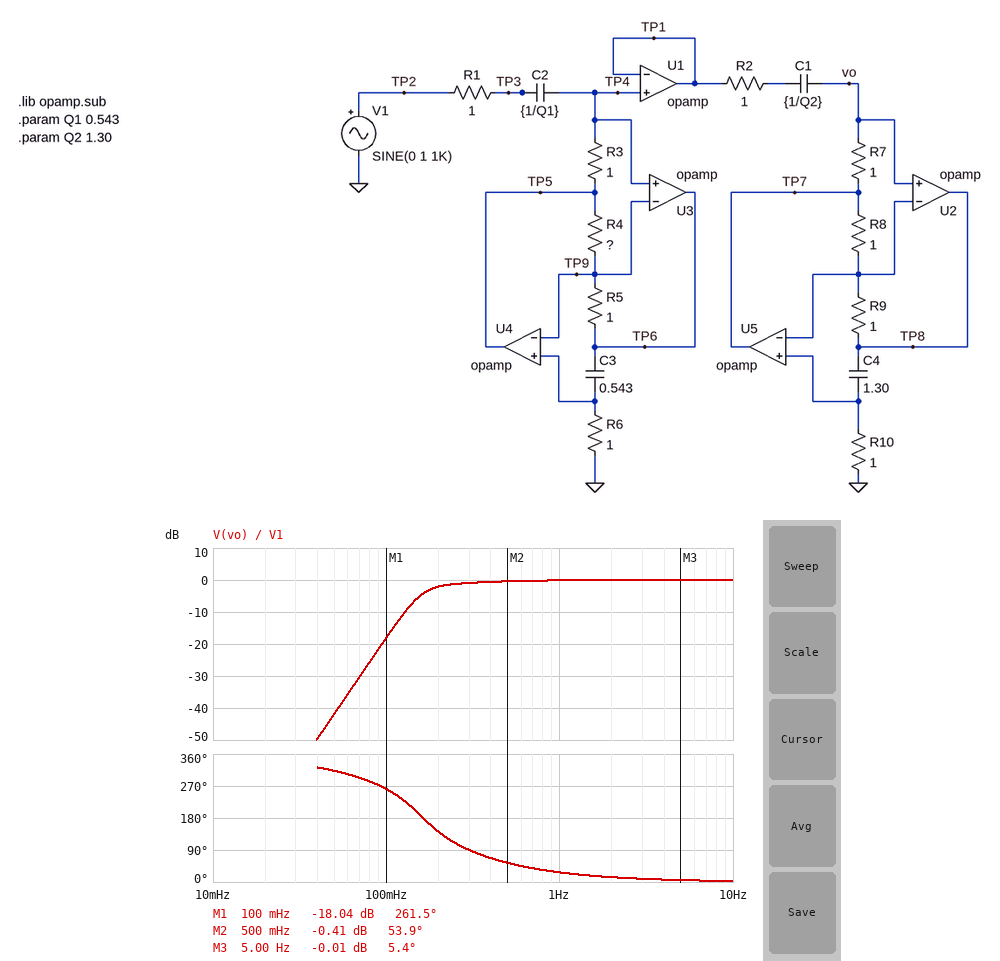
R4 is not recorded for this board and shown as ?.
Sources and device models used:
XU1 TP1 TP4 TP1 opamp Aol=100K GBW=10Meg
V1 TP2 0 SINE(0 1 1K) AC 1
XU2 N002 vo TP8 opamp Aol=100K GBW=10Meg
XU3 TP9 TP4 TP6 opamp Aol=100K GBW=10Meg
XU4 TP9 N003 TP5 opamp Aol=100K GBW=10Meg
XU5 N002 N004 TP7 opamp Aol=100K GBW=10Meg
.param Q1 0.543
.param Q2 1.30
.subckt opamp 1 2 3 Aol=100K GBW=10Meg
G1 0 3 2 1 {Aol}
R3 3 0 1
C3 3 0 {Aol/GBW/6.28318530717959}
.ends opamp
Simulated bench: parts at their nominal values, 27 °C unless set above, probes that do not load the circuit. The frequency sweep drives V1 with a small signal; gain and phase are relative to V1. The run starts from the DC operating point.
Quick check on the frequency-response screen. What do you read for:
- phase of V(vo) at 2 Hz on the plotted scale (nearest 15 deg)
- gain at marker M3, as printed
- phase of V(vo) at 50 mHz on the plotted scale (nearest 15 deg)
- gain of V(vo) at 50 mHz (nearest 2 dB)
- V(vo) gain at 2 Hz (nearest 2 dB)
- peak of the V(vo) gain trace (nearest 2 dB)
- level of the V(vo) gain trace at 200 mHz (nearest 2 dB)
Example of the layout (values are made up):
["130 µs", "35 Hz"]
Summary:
["15 deg", "-0.01 dB", "315 deg", "-42 dB", "0 dB", "0 dB", "-2 dB"]
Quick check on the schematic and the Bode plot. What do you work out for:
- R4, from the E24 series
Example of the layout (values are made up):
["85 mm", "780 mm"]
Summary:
["1.2 Ω"]
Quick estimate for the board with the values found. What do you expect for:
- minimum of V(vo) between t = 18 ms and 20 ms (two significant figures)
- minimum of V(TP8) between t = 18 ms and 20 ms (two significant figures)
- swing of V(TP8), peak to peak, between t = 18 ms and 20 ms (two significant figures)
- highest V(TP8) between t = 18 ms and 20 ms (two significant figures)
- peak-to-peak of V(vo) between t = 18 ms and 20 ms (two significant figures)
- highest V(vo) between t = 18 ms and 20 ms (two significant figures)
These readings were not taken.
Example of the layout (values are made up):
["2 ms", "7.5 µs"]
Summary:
["-1.0 V", "-1.0 V", "2.0 V", "1.0 V", "2.0 V", "1.0 V"]
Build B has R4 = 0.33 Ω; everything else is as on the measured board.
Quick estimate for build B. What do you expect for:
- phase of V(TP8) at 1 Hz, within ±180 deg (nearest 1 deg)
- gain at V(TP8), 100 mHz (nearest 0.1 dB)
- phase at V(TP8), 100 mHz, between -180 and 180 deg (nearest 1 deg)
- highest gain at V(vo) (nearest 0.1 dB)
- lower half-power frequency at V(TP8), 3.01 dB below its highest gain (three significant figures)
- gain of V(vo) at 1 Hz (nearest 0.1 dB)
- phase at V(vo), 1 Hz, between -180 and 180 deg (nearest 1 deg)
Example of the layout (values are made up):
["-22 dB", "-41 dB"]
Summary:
["6 deg", "-1.7 dB", "171 deg", "3.7 dB", "124 mHz", "0.2 dB", "13 deg"]
